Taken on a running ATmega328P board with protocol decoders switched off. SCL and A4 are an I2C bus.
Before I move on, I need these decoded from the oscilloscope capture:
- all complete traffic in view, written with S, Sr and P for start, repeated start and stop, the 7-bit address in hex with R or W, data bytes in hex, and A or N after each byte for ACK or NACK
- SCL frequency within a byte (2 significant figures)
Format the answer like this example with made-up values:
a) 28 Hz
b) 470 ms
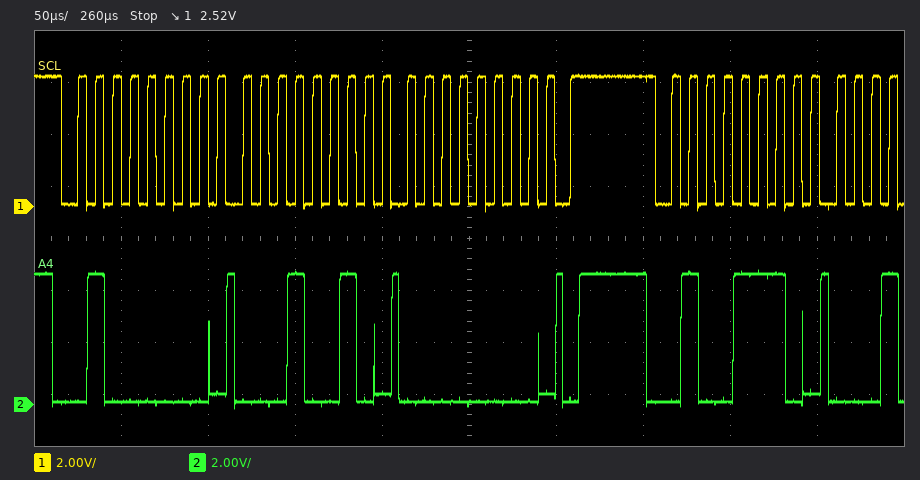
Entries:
a) S 20W A 12 A 00 A P S 27W A
b) 100 kHz
